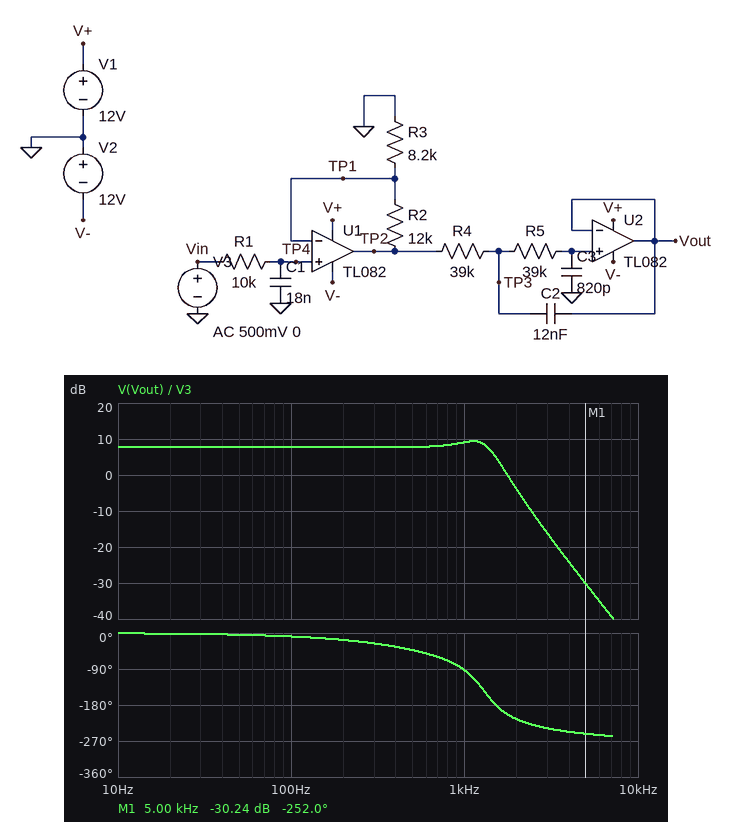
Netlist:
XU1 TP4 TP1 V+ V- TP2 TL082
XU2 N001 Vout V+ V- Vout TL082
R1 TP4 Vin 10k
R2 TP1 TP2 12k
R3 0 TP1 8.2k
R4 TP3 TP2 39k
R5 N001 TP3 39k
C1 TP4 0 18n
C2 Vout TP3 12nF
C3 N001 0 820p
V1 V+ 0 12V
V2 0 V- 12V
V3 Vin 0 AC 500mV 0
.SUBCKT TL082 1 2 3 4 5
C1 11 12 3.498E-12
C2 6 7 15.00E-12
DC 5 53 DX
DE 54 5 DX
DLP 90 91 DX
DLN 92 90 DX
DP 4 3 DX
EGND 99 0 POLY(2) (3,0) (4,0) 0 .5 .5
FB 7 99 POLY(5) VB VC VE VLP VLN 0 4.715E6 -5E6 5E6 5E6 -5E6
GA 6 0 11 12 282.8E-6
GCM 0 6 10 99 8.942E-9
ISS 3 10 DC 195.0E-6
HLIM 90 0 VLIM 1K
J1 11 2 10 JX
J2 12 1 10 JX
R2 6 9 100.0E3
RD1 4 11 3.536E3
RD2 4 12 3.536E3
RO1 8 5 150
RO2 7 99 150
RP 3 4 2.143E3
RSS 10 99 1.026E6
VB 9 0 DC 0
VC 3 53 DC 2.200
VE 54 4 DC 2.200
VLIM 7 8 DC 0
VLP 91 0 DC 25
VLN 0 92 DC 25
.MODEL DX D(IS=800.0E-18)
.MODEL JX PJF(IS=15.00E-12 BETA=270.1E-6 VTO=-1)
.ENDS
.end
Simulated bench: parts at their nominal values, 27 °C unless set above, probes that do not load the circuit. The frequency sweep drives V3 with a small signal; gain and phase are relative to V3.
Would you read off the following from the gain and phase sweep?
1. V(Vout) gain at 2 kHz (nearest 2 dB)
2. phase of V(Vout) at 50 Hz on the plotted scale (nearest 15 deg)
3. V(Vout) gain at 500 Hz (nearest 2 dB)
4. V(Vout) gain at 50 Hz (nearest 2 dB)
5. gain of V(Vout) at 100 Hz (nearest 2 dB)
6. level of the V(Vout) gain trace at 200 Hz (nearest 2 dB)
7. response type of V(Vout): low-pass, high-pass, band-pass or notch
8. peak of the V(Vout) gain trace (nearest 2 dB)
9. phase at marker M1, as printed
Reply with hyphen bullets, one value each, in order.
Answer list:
- -4 dB
- 0 deg
- 8 dB
- 8 dB
- 8 dB
- 8 dB
- low-pass
- 10 dB
- -252.0 deg
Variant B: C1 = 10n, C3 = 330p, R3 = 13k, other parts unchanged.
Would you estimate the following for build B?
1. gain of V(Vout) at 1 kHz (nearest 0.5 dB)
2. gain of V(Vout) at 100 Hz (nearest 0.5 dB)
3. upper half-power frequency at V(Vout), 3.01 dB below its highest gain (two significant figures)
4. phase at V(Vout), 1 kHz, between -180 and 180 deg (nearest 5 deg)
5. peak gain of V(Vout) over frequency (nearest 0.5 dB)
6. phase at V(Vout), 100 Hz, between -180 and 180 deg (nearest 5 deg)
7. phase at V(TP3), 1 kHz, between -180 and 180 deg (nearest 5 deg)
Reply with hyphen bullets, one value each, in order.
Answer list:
- 6.5 dB
- 5.5 dB
- 2.3 kHz
- -45 deg
- 11.5 dB
- -5 deg
- -40 deg
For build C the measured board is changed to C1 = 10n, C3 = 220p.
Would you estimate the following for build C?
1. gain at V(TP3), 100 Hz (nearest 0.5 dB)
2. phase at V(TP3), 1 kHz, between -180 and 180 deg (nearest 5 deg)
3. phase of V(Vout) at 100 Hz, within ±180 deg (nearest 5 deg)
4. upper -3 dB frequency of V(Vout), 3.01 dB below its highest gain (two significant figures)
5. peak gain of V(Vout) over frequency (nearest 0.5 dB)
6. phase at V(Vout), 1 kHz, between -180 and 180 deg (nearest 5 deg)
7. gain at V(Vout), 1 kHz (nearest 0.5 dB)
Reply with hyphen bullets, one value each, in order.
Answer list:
- 8.0 dB
- -35 deg
- -5 deg
- 2.7 kHz
- 14.0 dB
- -40 deg
- 8.0 dB
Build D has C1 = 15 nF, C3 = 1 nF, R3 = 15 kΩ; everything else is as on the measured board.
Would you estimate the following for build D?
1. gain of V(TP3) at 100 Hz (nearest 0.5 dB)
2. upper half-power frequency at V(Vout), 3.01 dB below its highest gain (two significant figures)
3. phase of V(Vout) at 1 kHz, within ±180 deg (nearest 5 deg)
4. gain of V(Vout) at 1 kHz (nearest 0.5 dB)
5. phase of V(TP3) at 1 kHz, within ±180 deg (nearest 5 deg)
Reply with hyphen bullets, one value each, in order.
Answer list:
- 5.0 dB
- 1.3 kHz
- -105 deg
- 7.5 dB
- -90 deg
